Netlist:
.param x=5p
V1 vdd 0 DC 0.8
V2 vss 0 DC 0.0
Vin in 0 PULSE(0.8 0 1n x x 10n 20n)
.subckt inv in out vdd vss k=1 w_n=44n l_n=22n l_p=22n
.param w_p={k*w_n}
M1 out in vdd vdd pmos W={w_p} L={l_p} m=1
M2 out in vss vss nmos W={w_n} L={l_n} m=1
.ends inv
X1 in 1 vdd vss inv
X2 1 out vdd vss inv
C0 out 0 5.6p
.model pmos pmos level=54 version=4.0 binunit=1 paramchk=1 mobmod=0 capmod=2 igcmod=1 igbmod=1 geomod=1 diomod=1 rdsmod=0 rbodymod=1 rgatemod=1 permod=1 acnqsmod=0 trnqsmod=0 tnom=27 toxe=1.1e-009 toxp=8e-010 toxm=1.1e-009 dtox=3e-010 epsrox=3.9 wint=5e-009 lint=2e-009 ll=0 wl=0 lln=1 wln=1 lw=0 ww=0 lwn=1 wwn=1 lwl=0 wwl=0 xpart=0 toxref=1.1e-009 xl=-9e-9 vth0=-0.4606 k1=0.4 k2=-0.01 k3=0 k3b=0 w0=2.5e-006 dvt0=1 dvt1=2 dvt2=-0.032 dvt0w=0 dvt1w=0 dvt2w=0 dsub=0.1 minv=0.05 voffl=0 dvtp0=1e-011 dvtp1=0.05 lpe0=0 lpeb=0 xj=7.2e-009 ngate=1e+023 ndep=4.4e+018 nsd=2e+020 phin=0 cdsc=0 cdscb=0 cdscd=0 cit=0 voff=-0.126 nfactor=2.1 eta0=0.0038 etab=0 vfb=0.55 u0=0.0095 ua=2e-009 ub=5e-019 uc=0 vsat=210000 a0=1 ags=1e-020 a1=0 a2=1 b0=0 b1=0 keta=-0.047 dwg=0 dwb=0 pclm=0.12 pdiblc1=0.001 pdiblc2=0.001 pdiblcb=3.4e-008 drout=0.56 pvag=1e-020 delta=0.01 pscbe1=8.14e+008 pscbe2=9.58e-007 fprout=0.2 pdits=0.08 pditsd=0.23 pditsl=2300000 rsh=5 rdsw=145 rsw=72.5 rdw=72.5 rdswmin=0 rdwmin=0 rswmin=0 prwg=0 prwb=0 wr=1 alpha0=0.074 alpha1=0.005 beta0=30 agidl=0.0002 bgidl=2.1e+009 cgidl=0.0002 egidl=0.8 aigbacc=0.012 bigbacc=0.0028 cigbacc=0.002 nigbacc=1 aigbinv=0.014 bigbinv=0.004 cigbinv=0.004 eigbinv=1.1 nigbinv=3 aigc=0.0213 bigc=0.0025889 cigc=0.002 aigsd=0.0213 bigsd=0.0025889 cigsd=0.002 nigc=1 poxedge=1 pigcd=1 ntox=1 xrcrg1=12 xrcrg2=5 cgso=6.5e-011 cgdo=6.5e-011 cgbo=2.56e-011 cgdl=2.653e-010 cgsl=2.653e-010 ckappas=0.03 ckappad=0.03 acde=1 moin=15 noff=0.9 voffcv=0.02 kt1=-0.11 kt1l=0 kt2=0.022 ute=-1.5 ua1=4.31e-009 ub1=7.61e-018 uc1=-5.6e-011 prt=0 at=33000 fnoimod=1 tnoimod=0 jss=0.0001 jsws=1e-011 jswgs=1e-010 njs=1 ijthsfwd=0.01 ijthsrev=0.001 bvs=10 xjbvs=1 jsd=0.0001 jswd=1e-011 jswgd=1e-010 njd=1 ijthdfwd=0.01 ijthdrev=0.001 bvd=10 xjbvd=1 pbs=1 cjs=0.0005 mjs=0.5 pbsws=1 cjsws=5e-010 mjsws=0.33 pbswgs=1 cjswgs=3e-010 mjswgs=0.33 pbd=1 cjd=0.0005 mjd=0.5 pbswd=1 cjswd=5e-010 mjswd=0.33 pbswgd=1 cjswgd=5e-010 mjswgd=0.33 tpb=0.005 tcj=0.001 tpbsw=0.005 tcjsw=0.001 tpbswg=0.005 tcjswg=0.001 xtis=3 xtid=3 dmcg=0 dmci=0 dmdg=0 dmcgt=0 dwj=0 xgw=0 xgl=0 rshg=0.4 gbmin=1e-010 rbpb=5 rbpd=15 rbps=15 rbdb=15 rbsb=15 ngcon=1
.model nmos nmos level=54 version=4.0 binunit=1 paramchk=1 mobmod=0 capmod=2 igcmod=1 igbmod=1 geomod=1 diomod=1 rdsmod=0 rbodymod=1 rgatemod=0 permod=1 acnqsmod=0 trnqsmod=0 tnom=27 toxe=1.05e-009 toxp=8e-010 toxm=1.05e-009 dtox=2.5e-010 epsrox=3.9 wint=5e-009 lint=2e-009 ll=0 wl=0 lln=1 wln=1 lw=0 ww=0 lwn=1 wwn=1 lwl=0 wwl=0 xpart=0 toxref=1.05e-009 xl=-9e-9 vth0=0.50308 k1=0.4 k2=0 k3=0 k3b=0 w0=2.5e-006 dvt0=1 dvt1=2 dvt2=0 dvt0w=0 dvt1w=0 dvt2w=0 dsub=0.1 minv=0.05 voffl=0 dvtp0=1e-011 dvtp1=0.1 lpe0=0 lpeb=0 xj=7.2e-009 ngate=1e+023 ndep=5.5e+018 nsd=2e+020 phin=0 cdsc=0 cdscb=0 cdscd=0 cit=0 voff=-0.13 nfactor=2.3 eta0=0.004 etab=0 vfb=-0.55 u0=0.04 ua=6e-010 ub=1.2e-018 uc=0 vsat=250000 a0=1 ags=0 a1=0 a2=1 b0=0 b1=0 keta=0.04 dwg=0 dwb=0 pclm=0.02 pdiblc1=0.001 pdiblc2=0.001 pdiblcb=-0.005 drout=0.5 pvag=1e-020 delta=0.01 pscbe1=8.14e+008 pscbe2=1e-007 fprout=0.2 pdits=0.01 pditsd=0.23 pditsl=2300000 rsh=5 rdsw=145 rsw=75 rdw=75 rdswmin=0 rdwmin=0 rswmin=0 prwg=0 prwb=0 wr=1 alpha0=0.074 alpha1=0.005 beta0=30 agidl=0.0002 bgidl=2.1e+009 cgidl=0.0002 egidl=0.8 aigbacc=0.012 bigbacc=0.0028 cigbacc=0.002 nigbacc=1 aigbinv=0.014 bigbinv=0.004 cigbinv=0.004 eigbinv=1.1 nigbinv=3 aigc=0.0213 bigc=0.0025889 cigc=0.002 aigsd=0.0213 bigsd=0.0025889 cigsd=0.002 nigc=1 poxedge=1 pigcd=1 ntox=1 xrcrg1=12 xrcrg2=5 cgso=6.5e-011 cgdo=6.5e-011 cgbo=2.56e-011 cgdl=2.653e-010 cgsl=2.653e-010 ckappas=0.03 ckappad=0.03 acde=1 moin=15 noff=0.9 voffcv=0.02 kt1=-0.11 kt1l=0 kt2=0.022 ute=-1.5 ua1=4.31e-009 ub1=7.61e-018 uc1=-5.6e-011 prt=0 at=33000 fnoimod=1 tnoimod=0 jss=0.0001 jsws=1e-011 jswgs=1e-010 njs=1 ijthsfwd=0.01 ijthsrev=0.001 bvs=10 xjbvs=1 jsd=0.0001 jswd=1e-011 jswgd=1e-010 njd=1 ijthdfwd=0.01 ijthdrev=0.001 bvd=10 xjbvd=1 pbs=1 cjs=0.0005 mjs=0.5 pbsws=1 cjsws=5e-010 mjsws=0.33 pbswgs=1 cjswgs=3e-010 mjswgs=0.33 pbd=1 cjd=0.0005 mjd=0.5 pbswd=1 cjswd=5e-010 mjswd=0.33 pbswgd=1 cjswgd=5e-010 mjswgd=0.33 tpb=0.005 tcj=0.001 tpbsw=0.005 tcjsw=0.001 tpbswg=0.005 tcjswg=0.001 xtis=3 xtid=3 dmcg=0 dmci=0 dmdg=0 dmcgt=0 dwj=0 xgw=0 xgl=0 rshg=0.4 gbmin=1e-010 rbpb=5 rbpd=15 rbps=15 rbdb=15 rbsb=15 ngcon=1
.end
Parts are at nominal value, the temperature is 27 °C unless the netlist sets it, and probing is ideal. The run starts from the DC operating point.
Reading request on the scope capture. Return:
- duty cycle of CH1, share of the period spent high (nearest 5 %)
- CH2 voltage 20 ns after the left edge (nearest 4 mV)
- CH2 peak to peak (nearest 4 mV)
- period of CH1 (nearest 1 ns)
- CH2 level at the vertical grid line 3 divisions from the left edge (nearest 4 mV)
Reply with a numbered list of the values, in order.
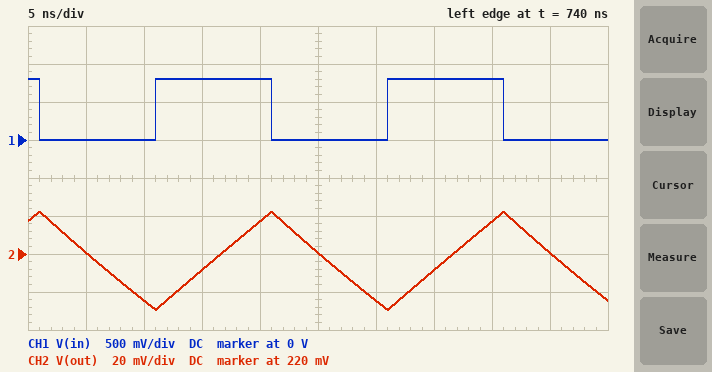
1. 50 %
2. 236 mV
3. 52 mV
4. 20 ns
5. 212 mV
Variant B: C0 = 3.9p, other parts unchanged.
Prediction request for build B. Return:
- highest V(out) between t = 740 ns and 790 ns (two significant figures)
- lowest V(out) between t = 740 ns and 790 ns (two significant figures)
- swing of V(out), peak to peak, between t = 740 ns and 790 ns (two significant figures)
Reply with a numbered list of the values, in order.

1. 250 mV
2. 180 mV
3. 74 mV
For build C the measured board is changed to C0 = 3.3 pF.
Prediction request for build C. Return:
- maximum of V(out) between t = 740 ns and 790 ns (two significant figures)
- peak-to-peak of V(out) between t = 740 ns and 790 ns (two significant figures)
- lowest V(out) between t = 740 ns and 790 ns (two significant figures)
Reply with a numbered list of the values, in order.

1. 260 mV
2. 87 mV
3. 170 mV
